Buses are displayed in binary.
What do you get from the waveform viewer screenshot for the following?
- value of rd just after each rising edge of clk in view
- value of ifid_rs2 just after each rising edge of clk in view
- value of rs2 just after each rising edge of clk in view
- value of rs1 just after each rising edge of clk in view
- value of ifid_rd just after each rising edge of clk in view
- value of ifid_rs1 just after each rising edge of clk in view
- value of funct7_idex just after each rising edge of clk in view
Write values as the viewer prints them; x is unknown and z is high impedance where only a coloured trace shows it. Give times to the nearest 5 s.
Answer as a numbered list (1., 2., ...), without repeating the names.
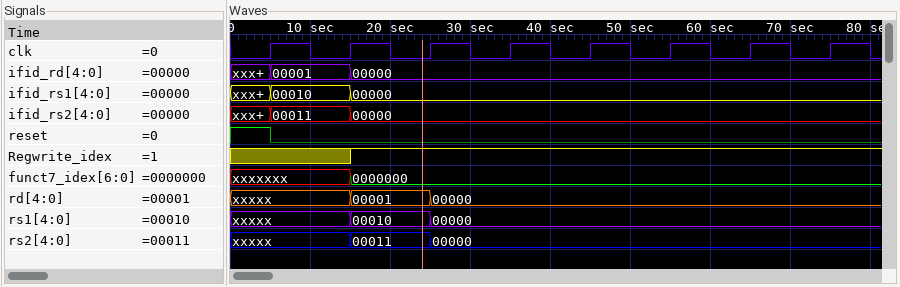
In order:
1. xxxxx, 00001, 00000, 00000, 00000, 00000, 00000, 00000
2. 00011, 00000, 00000, 00000, 00000, 00000, 00000, 00000
3. xxxxx, 00011, 00000, 00000, 00000, 00000, 00000, 00000
4. xxxxx, 00010, 00000, 00000, 00000, 00000, 00000, 00000
5. 00001, 00000, 00000, 00000, 00000, 00000, 00000, 00000
6. 00010, 00000, 00000, 00000, 00000, 00000, 00000, 00000
7. xxxxxxx, 0000000, 0000000, 0000000, 0000000, 0000000, 0000000, 0000000
